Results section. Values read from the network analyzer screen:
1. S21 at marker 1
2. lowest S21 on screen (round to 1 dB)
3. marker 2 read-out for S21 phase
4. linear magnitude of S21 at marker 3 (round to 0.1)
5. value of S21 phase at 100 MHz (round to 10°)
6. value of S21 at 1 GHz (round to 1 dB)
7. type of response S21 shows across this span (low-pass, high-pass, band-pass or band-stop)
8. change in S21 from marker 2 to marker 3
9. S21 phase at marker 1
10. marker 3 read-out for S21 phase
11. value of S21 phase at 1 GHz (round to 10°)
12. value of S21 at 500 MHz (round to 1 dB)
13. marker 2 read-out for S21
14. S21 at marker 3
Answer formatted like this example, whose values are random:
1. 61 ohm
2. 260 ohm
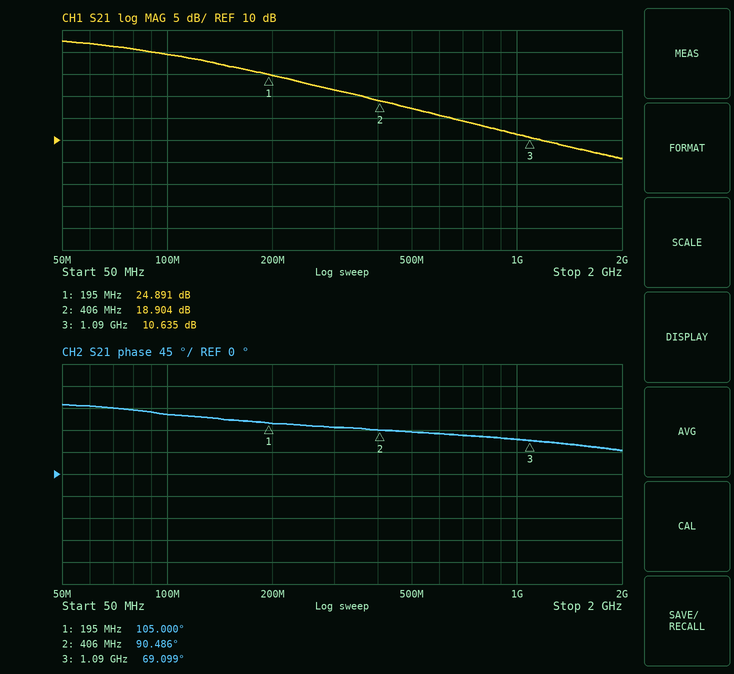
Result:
1. 24.891 dB
2. 6 dB
3. 90.486°
4. 3.4
5. 120°
6. 11 dB
7. low-pass
8. -8.269 dB
9. 105.000°
10. 69.099°
11. 70°
12. 17 dB
13. 18.904 dB
14. 10.635 dB
